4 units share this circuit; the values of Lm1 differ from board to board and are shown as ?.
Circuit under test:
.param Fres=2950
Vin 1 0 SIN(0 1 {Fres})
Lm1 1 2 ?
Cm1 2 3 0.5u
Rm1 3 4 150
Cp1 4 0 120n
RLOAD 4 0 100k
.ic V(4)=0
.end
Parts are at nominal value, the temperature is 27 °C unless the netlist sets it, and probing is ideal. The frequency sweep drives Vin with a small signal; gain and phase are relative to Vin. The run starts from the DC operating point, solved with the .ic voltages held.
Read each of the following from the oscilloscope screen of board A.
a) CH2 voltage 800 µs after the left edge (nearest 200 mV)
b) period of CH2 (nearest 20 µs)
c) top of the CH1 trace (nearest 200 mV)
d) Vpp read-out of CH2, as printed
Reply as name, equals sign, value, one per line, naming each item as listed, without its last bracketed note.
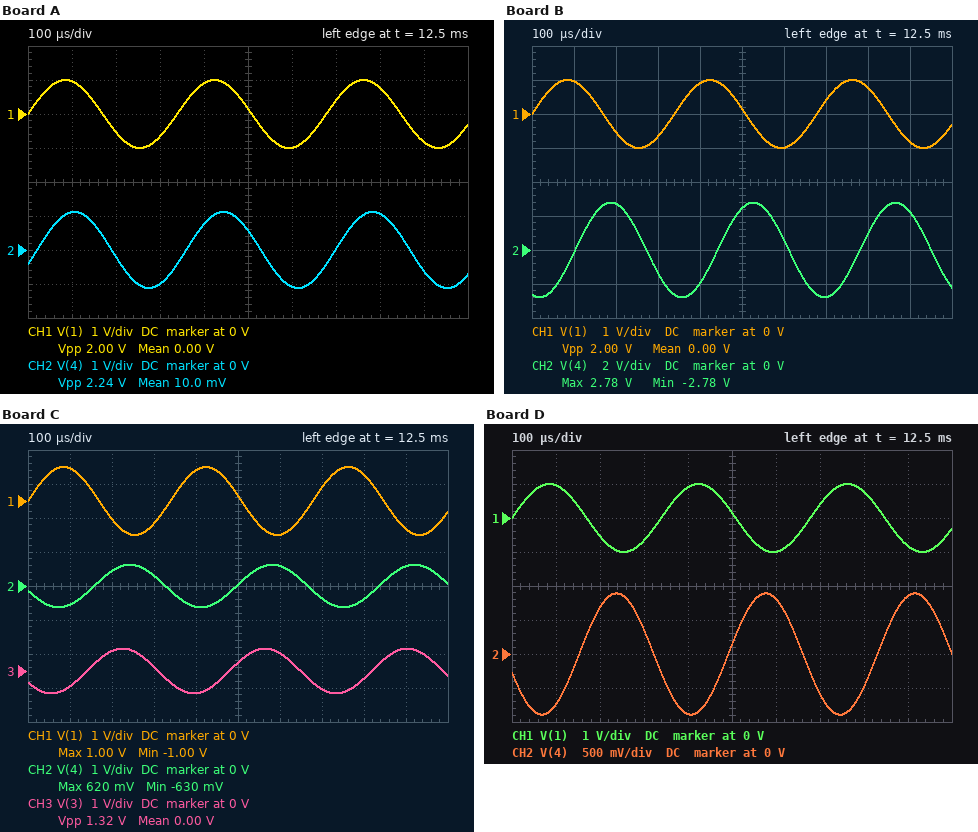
CH2 voltage 800 µs after the left edge = 1.0 V
period of CH2 = 340 µs
top of the CH1 trace = 1.0 V
Vpp read-out of CH2, as printed = 2.24 V
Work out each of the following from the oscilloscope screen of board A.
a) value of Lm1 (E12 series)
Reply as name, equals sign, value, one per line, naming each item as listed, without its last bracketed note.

value of Lm1 = 10 mH
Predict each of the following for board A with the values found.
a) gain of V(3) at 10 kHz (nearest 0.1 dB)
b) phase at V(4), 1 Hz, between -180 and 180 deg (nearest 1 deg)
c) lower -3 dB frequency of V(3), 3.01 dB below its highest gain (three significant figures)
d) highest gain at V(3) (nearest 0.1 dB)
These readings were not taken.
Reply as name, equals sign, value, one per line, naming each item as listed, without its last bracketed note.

gain of V(3) at 10 kHz = -7.7 dB
phase at V(4), 1 Hz, between -180 and 180 deg = 69 deg
lower -3 dB frequency of V(3), 3.01 dB below its highest gain = 3.57 kHz
highest gain at V(3) = 6.1 dB
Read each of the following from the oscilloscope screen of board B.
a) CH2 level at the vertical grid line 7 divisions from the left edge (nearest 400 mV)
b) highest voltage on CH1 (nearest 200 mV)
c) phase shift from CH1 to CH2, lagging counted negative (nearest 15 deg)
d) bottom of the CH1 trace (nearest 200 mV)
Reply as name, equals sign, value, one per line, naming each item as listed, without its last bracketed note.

CH2 level at the vertical grid line 7 divisions from the left edge = -2.8 V
highest voltage on CH1 = 1.0 V
phase shift from CH1 to CH2, lagging counted negative = -105 deg
bottom of the CH1 trace = -1.0 V
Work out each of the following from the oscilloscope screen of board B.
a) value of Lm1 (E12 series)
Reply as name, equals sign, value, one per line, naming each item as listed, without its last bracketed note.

value of Lm1 = 33 mH
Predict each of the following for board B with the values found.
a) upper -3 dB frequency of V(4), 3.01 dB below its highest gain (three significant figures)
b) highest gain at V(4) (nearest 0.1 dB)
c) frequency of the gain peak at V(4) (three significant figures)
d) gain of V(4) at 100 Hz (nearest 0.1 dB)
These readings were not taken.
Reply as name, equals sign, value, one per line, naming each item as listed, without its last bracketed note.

upper -3 dB frequency of V(4), 3.01 dB below its highest gain = 3.12 kHz
highest gain at V(4) = 9.9 dB
frequency of the gain peak at V(4) = 2.77 kHz
gain of V(4) at 100 Hz = -1.9 dB
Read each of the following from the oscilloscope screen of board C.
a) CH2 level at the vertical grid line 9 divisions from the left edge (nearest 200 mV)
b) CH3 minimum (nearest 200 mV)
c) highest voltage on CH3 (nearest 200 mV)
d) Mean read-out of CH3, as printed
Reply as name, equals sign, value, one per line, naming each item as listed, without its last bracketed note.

CH2 level at the vertical grid line 9 divisions from the left edge = 600 mV
CH3 minimum = -600 mV
highest voltage on CH3 = 600 mV
Mean read-out of CH3, as printed = 0.00 V
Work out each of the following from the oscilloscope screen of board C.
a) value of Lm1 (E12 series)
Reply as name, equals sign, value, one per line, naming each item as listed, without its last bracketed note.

value of Lm1 = 68 mH
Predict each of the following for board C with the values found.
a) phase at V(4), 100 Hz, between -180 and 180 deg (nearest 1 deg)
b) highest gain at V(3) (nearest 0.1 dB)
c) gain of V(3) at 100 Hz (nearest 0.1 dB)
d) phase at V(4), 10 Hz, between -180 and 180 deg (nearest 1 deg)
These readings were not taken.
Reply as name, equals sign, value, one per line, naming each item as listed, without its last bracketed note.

phase at V(4), 100 Hz, between -180 and 180 deg = 1 deg
highest gain at V(3) = 13.1 dB
gain of V(3) at 100 Hz = -1.8 dB
phase at V(4), 10 Hz, between -180 and 180 deg = 14 deg
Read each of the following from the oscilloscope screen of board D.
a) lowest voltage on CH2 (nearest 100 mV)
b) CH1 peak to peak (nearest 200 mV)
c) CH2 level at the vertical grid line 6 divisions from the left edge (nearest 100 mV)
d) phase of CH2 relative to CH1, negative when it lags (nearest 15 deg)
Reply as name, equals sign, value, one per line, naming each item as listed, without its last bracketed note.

lowest voltage on CH2 = -900 mV
CH1 peak to peak = 2.0 V
CH2 level at the vertical grid line 6 divisions from the left edge = 800 mV
phase of CH2 relative to CH1, negative when it lags = -165 deg
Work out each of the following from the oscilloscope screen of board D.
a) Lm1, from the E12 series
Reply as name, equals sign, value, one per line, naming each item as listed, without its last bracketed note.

Lm1, from the E12 series = 56 mH
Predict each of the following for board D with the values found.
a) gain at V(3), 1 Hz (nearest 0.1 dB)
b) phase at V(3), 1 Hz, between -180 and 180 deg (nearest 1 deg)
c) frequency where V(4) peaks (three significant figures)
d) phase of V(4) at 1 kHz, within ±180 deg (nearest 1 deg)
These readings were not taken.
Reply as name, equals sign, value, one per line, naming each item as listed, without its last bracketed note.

gain at V(3), 1 Hz = -10.7 dB
phase at V(3), 1 Hz, between -180 and 180 deg = 69 deg
frequency where V(4) peaks = 2.14 kHz
phase of V(4) at 1 kHz, within ±180 deg = -7 deg
